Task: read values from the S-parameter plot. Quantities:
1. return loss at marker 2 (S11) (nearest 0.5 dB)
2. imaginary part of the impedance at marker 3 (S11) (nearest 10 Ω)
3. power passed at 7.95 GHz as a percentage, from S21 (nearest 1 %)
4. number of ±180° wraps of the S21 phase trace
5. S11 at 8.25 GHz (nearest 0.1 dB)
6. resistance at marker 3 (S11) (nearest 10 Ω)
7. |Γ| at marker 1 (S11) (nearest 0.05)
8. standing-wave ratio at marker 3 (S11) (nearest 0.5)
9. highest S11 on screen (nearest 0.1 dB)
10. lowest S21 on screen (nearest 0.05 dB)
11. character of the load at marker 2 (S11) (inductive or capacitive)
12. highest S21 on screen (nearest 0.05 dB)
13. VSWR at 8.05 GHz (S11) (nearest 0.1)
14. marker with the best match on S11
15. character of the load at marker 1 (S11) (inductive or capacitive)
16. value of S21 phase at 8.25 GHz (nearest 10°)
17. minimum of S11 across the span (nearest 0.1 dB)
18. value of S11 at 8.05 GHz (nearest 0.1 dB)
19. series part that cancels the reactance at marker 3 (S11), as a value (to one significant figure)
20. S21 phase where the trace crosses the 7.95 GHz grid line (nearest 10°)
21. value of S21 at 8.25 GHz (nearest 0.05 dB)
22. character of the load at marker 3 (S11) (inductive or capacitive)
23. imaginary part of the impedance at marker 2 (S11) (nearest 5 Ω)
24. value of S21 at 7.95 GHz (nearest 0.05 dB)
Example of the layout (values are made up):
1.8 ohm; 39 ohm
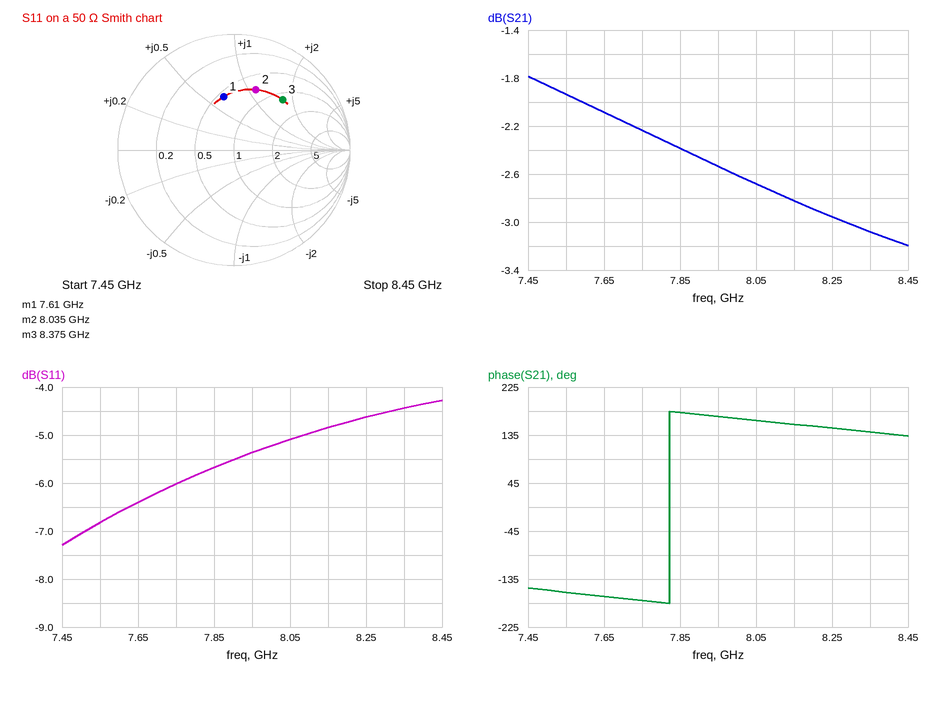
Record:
5.0 dB; +80 Ω; 56 %; 1; -4.6 dB; 60 Ω; 0.45; 4.0; -4.3 dB; -3.20 dB; inductive; -1.80 dB; 3.5; marker 1; inductive; 150°; -7.3 dB; -5.1 dB; 200 fF; 170°; -2.95 dB; inductive; +55 Ω; -2.55 dB
